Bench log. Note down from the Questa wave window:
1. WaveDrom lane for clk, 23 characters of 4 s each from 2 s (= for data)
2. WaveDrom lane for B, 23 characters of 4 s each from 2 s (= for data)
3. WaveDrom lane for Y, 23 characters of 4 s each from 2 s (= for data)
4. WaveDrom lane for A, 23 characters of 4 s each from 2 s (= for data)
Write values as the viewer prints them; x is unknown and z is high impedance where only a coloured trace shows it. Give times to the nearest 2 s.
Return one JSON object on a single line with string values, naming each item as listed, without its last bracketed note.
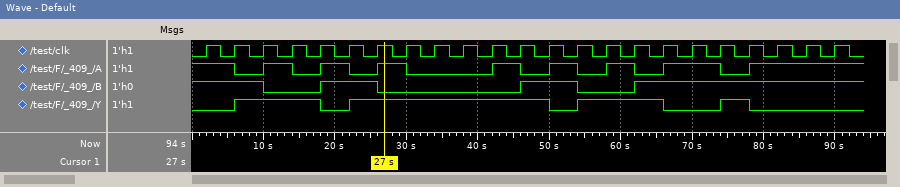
{"WaveDrom lane for clk, 23 characters of 4 s each from 2 s": "{name: 'clk', wave: 'p......................'}", "WaveDrom lane for B, 23 characters of 4 s each from 2 s": "{name: 'B', wave: '1.0.1.0....1.0.1.......'}", "WaveDrom lane for Y, 23 characters of 4 s each from 2 s": "{name: 'Y', wave: '01..01......01..0.10...'}", "WaveDrom lane for A, 23 characters of 4 s each from 2 s": "{name: 'A', wave: '10101010..1010101.01...'}"}
